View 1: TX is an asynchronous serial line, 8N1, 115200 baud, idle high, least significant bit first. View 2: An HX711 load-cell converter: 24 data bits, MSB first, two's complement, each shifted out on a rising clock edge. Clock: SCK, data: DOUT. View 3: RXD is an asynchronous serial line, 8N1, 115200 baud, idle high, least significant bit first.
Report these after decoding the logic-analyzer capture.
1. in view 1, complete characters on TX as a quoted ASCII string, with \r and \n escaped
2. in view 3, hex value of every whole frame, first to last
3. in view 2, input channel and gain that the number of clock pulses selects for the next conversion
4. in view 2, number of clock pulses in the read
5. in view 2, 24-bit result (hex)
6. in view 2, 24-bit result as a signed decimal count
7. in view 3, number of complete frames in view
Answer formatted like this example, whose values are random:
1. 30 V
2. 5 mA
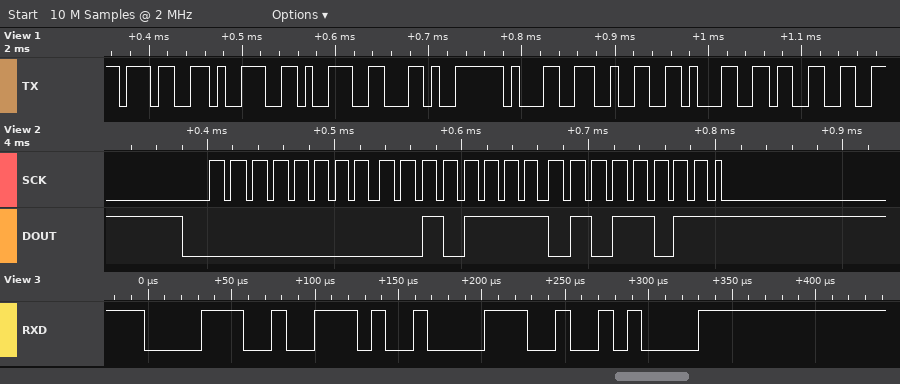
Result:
1. "799,1213"
2. 38 2E 38 0A
3. channel A, gain 128
4. 25
5. 0x002F5B
6. 12123
7. 4
